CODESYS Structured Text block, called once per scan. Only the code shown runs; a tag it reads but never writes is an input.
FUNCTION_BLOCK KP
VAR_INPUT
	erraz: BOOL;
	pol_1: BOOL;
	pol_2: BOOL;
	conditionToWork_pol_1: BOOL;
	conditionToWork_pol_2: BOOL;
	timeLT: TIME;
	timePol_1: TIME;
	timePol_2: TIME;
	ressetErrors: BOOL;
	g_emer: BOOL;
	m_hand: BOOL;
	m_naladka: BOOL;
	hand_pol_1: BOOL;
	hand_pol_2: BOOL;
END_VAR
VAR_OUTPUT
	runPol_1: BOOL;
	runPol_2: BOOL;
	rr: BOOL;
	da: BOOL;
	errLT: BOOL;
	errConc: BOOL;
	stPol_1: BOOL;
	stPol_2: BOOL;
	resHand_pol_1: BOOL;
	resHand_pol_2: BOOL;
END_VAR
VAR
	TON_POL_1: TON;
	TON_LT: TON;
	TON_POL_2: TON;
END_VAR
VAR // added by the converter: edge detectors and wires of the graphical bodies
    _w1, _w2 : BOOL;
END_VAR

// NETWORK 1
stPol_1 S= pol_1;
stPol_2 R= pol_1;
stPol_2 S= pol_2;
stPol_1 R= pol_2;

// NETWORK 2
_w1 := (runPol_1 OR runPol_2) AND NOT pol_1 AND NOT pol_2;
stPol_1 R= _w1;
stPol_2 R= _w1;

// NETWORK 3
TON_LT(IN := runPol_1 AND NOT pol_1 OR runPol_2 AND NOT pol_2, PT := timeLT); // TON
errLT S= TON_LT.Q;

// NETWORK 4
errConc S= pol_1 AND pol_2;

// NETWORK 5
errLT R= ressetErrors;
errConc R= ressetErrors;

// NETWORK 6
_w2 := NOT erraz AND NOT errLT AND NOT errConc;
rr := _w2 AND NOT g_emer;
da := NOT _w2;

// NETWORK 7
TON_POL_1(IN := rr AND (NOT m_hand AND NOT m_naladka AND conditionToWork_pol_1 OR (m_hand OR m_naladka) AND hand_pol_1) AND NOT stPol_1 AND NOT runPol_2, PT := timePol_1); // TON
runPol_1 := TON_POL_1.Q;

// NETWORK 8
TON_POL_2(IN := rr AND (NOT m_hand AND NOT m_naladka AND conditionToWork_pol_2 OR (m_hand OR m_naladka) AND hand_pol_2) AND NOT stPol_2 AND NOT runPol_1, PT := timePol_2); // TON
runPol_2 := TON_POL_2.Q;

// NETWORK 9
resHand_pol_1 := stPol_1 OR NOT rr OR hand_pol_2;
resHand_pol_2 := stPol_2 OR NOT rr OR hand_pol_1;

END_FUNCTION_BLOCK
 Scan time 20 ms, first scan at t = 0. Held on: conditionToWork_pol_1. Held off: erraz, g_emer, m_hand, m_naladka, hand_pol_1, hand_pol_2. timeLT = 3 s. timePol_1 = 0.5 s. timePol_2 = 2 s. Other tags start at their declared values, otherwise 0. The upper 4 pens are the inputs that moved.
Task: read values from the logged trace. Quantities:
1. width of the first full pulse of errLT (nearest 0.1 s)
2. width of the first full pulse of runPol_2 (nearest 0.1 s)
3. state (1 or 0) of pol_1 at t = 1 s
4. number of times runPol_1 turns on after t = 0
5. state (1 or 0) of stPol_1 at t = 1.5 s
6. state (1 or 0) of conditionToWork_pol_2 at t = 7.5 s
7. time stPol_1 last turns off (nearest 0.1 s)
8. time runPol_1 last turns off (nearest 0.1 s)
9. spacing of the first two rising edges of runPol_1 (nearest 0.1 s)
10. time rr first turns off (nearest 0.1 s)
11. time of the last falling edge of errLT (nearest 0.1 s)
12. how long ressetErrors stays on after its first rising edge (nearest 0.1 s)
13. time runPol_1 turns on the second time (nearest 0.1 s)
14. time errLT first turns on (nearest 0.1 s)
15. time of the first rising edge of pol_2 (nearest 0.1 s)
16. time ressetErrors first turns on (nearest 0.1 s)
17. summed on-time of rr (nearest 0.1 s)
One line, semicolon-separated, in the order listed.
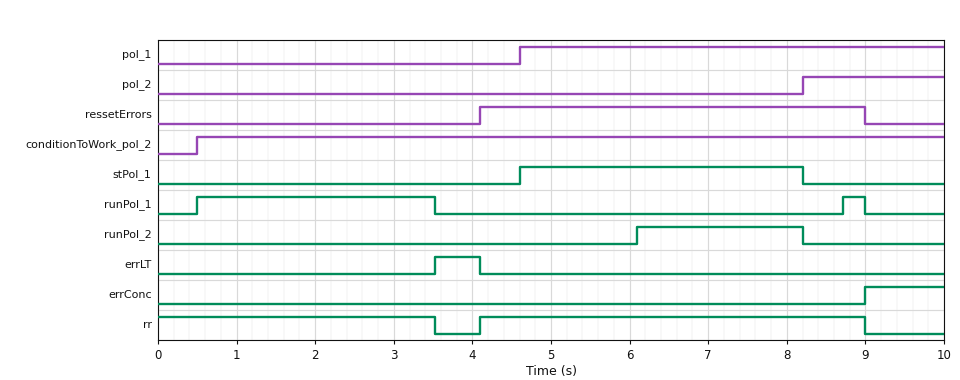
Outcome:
0.6 s; 2.1 s; 0; 2; 0; 1; 8.2 s; 9.0 s; 8.2 s; 3.5 s; 4.1 s; 4.9 s; 8.7 s; 3.5 s; 8.2 s; 4.1 s; 8.4 s
